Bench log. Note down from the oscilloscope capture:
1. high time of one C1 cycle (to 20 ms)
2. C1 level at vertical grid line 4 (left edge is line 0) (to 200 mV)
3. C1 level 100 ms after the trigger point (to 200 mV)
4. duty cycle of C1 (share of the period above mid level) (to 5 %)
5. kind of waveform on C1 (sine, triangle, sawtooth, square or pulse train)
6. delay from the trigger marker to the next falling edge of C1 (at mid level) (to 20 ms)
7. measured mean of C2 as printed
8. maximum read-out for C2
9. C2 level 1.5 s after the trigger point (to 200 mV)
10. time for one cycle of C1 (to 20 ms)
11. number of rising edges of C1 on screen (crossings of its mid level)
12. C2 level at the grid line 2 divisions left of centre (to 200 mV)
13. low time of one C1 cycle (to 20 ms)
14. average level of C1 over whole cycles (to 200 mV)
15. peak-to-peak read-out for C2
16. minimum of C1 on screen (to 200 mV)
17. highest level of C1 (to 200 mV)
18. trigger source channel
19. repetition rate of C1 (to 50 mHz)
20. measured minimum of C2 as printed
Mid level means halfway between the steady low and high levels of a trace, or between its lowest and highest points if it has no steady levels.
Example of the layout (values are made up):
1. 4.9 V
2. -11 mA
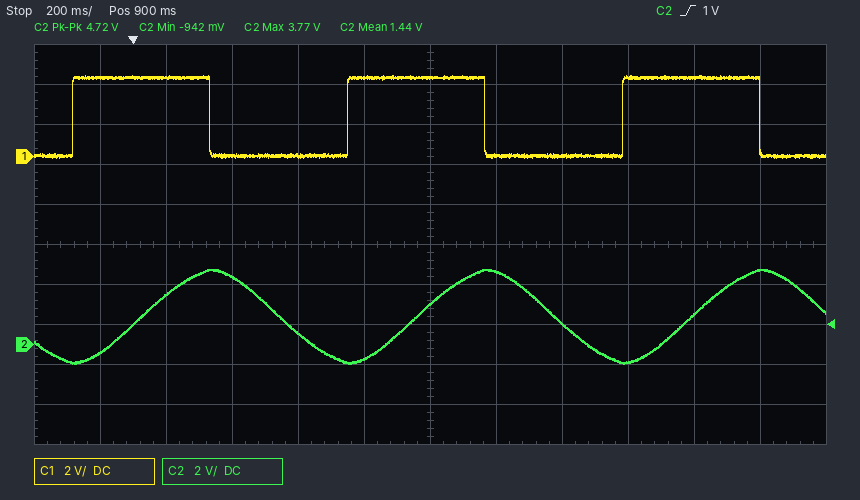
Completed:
1. 420 ms
2. 0.0 V
3. 4.0 V
4. 50 %
5. square
6. 240 ms
7. 1.44 V
8. 3.77 V
9. -800 mV
10. 840 ms
11. 3
12. 600 mV
13. 420 ms
14. 2.0 V
15. 4.72 V
16. 0.0 V
17. 4.0 V
18. C2
19. 1.20 Hz
20. -942 mV
